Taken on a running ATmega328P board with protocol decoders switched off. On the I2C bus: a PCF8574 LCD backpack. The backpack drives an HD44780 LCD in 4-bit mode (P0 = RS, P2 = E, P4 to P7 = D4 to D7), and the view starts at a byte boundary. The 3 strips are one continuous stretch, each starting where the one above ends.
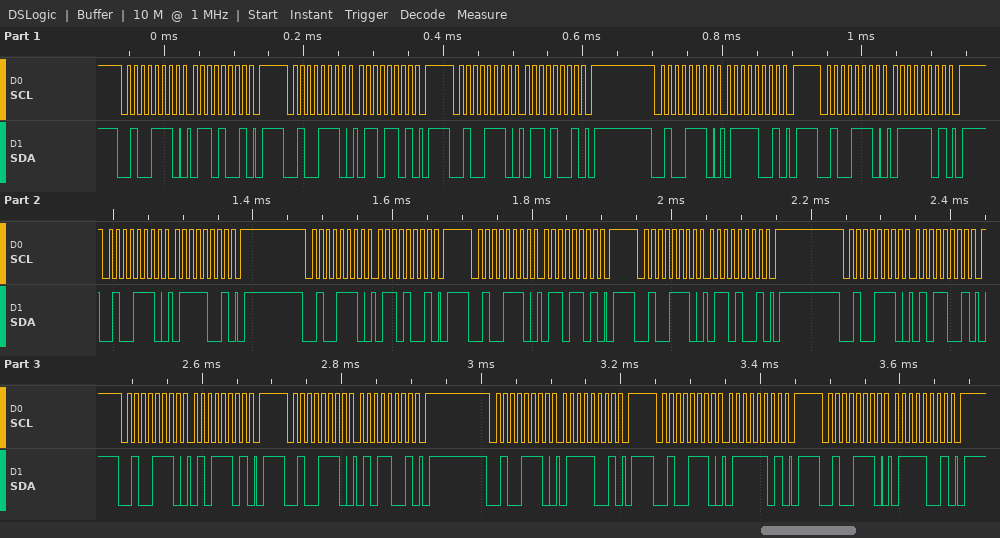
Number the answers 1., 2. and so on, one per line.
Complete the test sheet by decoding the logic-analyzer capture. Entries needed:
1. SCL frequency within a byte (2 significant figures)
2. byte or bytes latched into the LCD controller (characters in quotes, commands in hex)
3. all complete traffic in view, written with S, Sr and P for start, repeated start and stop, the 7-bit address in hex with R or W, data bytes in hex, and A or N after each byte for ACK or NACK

1. 100 kHz
2. 'g' 'e'
3. S 27W A 69 A P S 27W A 6D A P S 27W A 69 A P S 27W A 79 A P S 27W A 7D A P S 27W A 79 A P S 27W A 69 A P S 27W A 6D A P S 27W A 69 A P S 27W A 59 A P S 27W A 5D A P S 27W A 59 A P S 27W A 79 A P S 27W A 7D A P S 27W A 79 A P
